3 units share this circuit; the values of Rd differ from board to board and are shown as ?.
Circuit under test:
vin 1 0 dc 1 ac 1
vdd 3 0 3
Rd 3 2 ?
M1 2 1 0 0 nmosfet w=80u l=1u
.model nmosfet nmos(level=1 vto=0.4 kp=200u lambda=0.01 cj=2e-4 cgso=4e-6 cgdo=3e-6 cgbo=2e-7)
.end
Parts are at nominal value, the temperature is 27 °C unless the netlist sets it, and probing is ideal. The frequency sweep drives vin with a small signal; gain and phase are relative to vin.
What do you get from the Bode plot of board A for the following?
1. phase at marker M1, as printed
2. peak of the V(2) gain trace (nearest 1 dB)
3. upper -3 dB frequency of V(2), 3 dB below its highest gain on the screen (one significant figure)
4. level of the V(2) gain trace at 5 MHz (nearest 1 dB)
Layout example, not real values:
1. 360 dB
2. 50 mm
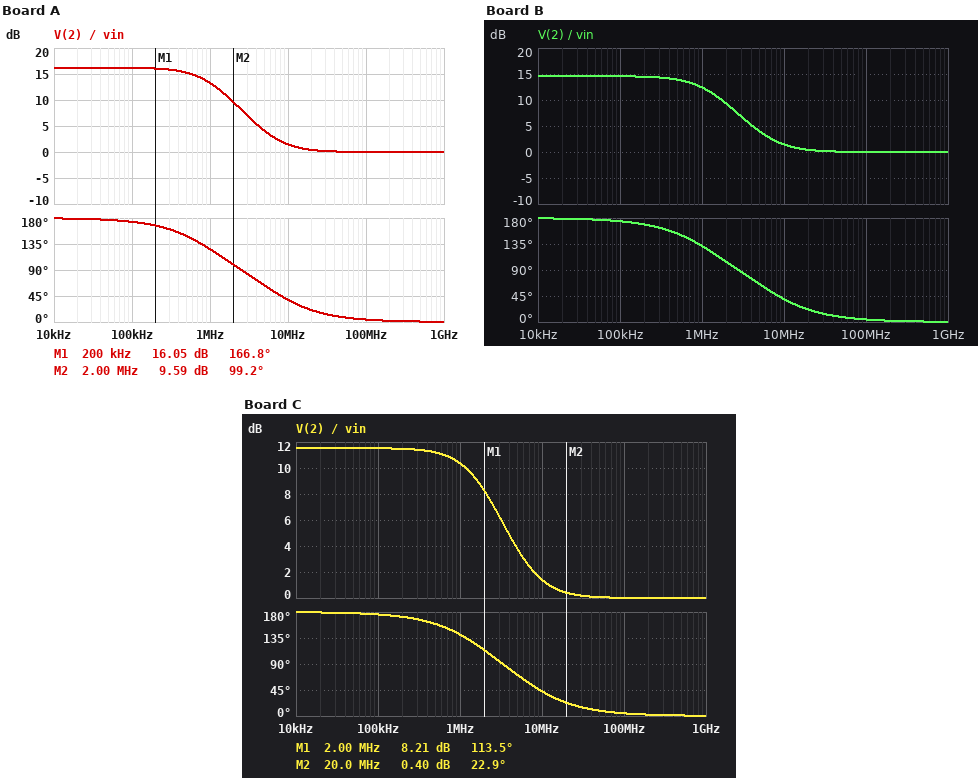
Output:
1. 166.8 deg
2. 16 dB
3. 1 MHz
4. 4 dB
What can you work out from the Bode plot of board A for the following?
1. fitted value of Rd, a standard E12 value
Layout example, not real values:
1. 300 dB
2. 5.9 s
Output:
1. 680 Ω
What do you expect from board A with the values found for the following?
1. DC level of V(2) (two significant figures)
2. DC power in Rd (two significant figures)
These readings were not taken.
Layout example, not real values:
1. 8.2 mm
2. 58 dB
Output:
1. 1.0 V
2. 5.8 mW
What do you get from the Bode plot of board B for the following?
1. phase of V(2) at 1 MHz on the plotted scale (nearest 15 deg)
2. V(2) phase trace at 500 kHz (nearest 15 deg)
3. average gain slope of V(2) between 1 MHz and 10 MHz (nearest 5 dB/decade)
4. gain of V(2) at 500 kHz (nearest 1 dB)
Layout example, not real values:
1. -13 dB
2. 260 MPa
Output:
1. 135 deg
2. 150 deg
3. -10 dB/decade
4. 14 dB
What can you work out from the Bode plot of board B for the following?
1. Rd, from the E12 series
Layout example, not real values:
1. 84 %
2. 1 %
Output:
1. 560 Ω
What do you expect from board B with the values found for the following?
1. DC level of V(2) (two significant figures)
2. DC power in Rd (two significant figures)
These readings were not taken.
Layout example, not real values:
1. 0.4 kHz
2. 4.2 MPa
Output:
1. 1.4 V
2. 4.8 mW
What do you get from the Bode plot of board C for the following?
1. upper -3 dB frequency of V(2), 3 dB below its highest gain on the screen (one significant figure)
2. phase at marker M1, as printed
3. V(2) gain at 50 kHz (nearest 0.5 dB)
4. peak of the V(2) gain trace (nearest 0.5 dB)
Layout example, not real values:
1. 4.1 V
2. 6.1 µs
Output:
1. 2 MHz
2. 113.5 deg
3. 11.5 dB
4. 11.5 dB
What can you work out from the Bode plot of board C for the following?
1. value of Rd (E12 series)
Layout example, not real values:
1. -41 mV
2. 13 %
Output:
1. 390 Ω
